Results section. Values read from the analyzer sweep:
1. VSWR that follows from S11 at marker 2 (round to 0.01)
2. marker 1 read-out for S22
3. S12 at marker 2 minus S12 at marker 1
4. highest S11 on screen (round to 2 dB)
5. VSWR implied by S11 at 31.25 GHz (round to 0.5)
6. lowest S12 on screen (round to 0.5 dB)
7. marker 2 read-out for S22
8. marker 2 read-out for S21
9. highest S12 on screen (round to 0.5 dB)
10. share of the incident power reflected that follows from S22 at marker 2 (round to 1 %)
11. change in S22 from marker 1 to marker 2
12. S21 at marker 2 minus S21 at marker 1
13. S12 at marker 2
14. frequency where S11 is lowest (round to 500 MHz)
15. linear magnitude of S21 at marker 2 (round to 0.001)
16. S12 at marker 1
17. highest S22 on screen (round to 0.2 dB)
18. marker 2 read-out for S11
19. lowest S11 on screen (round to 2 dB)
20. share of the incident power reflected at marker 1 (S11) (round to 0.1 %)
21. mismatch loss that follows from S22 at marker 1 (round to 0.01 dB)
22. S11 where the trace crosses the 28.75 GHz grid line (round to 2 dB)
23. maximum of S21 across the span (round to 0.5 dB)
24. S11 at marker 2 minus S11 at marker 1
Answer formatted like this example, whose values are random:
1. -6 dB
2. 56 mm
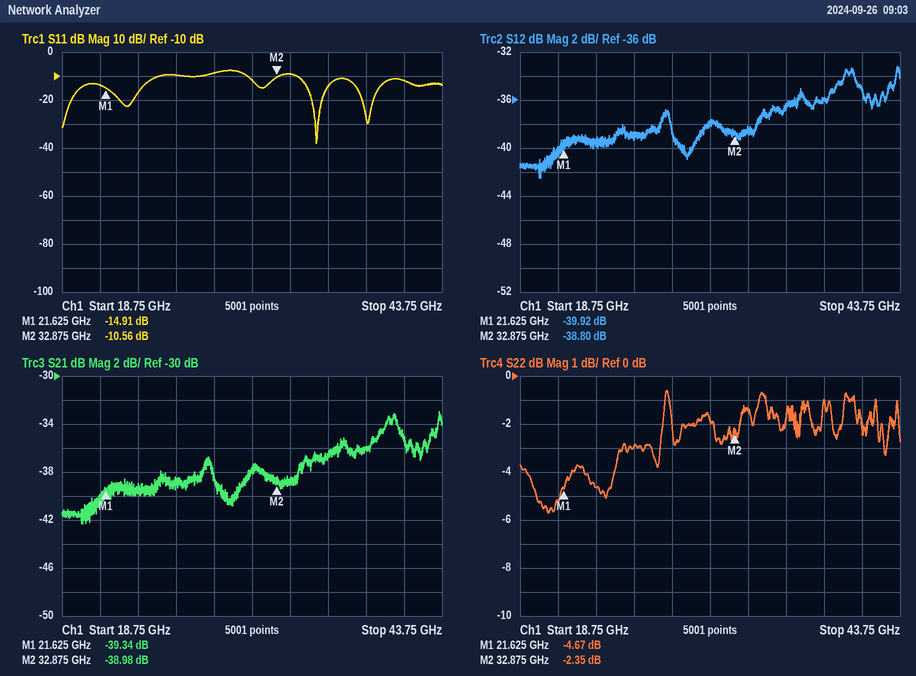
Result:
1. 1.84
2. -4.67 dB
3. 1.12 dB
4. -8 dB
5. 1.5
6. -42.5 dB
7. -2.35 dB
8. -38.98 dB
9. -33.0 dB
10. 58 %
11. 2.32 dB
12. 0.36 dB
13. -38.80 dB
14. 35.5 GHz
15. 0.011
16. -39.92 dB
17. -0.6 dB
18. -10.56 dB
19. -38 dB
20. 3.2 %
21. 1.81 dB
22. -8 dB
23. -33.0 dB
24. 4.35 dB
